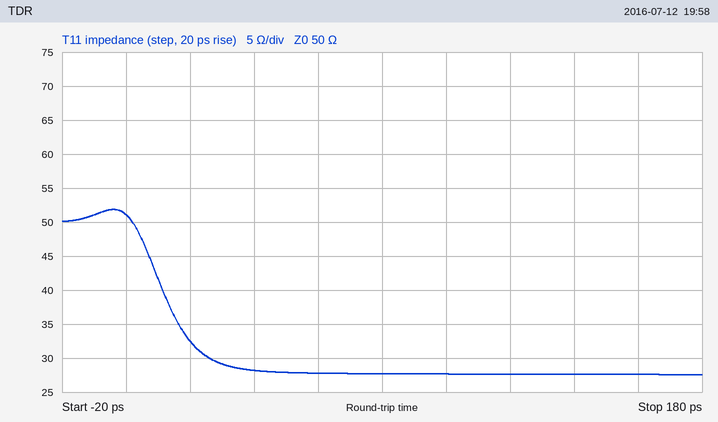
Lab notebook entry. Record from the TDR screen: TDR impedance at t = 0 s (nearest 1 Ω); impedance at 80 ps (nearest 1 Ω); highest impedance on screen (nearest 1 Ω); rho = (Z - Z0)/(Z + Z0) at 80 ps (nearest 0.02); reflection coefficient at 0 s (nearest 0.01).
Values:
51 Ω
28 Ω
52 Ω
-0.28
+0.01
